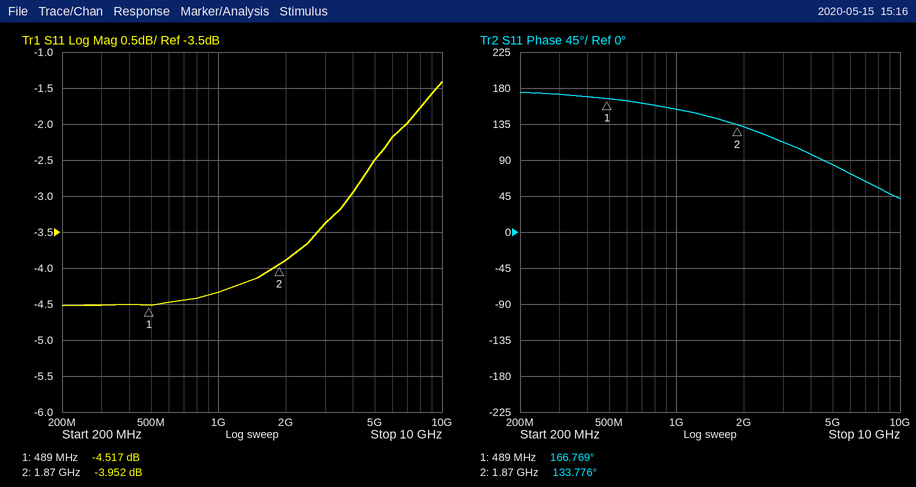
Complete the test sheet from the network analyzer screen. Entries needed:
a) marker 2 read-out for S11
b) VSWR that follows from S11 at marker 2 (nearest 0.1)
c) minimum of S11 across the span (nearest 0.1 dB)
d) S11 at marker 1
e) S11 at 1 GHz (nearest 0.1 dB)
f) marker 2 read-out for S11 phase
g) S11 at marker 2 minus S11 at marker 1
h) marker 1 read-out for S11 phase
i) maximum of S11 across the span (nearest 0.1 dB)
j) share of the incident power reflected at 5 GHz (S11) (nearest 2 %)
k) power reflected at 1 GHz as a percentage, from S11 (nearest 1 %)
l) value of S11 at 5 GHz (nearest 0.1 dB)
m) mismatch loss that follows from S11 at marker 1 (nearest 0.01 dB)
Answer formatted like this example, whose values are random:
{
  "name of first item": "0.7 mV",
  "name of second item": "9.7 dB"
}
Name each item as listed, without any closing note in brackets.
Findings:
{
  "marker 2 read-out for S11": "-3.952 dB",
  "VSWR that follows from S11 at marker 2": "4.5",
  "minimum of S11 across the span": "-4.5 dB",
  "S11 at marker 1": "-4.517 dB",
  "S11 at 1 GHz": "-4.3 dB",
  "marker 2 read-out for S11 phase": "133.776°",
  "S11 at marker 2 minus S11 at marker 1": "0.565 dB",
  "marker 1 read-out for S11 phase": "166.769°",
  "maximum of S11 across the span": "-1.4 dB",
  "share of the incident power reflected at 5 GHz (S11)": "56 %",
  "power reflected at 1 GHz as a percentage, from S11": "37 %",
  "value of S11 at 5 GHz": "-2.5 dB",
  "mismatch loss that follows from S11 at marker 1": "1.89 dB"
}
